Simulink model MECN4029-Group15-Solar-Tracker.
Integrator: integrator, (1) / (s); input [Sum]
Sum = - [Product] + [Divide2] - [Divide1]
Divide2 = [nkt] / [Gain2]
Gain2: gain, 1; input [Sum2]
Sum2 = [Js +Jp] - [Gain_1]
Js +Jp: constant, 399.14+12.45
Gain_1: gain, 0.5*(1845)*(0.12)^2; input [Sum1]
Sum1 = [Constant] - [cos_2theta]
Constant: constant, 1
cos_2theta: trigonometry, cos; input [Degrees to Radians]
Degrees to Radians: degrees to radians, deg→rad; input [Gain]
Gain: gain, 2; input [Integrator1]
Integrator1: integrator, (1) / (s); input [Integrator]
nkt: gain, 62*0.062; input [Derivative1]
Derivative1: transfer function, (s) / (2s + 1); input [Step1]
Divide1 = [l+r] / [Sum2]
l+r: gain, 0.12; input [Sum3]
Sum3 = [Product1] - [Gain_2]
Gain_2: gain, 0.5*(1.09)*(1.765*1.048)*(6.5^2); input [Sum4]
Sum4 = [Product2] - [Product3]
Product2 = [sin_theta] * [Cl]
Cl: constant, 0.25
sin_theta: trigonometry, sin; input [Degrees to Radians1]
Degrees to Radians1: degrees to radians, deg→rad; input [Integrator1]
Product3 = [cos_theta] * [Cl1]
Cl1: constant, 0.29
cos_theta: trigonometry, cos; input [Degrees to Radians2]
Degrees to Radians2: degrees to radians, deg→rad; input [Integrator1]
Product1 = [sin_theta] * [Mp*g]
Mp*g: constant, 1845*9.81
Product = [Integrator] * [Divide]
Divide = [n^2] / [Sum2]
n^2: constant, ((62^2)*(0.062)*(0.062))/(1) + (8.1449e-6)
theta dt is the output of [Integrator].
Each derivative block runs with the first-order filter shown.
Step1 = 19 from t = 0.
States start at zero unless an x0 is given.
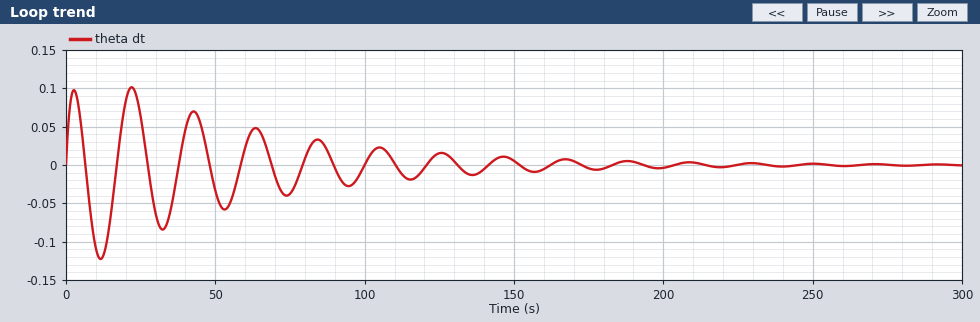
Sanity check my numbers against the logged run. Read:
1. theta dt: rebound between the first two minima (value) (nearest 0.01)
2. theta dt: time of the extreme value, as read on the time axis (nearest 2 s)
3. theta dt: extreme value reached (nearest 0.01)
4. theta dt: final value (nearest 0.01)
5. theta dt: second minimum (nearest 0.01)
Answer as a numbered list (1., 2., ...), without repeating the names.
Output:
1. 0.10
2. 12 s
3. -0.12
4. 0.00
5. -0.08
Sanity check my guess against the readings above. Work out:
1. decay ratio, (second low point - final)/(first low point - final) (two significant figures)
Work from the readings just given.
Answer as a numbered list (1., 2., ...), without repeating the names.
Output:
1. 0.67
